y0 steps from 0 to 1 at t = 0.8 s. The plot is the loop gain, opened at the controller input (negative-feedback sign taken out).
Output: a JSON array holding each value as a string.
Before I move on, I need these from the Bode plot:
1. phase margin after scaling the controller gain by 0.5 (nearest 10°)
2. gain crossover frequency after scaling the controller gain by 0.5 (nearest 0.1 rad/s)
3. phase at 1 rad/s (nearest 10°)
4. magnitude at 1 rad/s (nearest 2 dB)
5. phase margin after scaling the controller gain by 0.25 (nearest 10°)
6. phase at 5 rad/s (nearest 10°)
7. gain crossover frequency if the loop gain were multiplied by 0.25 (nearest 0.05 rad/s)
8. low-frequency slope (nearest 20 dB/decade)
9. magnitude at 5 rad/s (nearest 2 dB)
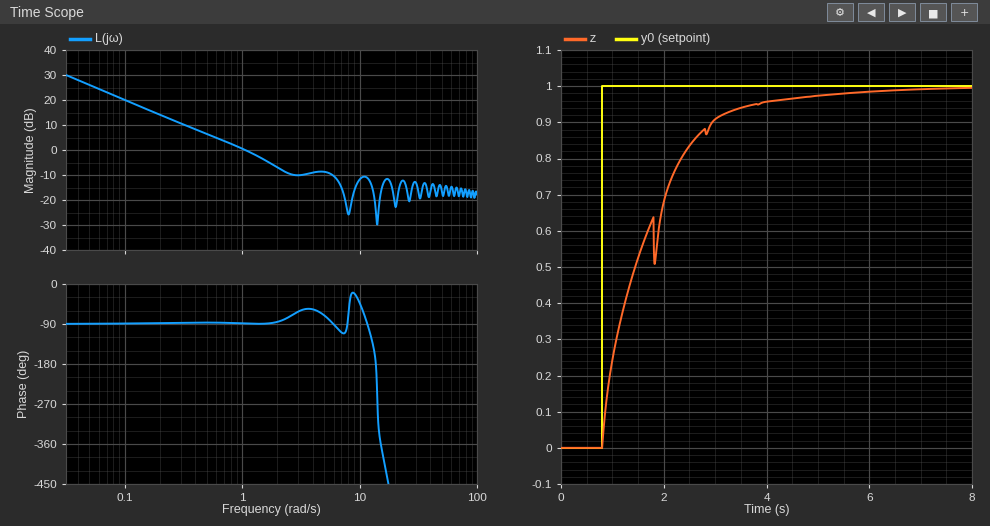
["90°", "0.5 rad/s", "-90°", "0 dB", "90°", "-70°", "0.25 rad/s", "-20 dB/decade", "-8 dB"]
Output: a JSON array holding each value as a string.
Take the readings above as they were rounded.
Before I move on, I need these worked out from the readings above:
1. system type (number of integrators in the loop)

["1"]
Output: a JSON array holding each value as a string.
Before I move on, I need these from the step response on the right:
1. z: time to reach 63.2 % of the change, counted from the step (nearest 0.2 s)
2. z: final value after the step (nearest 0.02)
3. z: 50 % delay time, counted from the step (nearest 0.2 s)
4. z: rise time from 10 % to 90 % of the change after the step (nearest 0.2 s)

["1.0 s", "1.00", "0.6 s", "2.0 s"]
